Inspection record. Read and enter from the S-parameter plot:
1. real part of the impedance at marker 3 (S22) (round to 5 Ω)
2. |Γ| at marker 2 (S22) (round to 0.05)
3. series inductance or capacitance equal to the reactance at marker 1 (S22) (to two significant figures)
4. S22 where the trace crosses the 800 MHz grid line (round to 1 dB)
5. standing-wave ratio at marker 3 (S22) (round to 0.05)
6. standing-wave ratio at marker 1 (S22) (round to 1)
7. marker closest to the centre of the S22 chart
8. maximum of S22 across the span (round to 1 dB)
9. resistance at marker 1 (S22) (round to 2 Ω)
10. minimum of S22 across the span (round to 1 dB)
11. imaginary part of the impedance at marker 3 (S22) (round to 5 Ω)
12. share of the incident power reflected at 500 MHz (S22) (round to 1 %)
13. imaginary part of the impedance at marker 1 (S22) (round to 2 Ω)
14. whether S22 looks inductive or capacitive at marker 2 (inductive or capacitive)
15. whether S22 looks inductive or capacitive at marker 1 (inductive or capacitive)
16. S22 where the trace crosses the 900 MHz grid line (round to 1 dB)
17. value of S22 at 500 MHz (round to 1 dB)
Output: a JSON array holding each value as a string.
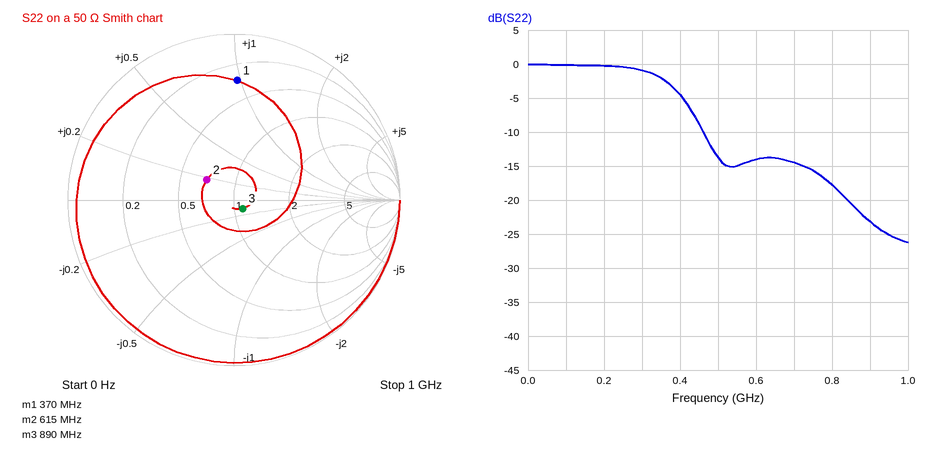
["55 Ω", "0.20", "21 nH", "-18 dB", "1.15", "6", "marker 3", "0 dB", "16 Ω", "-26 dB", "-5 Ω", "4 %", "+48 Ω", "inductive", "inductive", "-23 dB", "-14 dB"]
